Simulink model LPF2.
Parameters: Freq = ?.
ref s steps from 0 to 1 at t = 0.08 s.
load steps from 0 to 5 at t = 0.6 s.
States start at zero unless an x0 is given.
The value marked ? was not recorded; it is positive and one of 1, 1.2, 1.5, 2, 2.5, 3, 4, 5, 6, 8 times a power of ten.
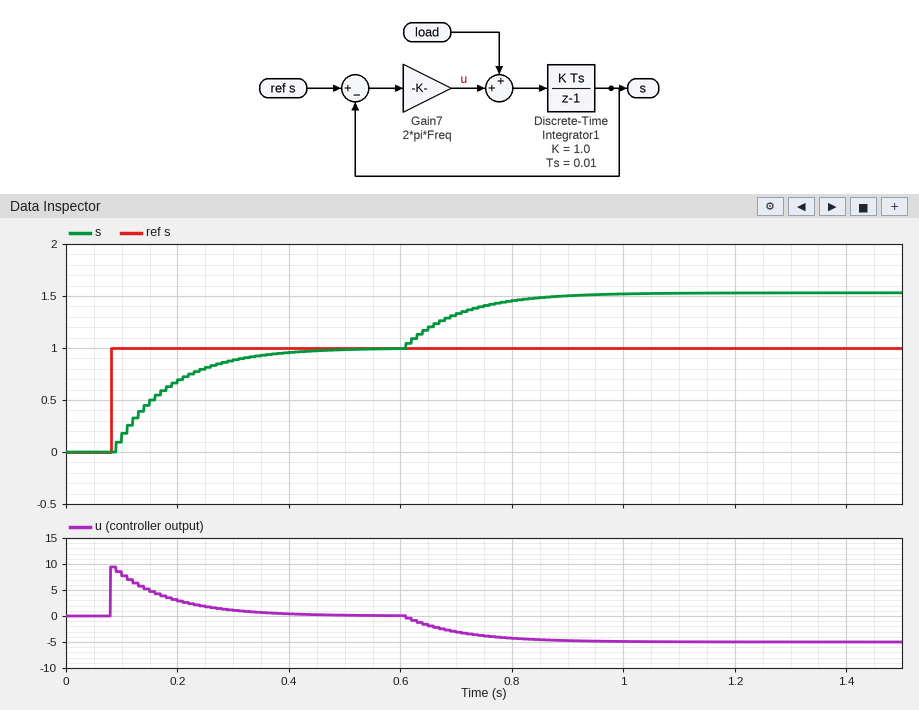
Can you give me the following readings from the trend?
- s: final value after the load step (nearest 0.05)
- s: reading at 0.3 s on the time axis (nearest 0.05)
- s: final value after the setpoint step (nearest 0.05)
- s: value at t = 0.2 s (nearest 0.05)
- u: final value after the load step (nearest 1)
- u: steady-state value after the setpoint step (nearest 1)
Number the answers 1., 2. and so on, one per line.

1. 1.55
2. 0.90
3. 1.00
4. 0.70
5. -5
6. 0
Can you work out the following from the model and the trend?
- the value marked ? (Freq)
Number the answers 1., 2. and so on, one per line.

1. 1.5
